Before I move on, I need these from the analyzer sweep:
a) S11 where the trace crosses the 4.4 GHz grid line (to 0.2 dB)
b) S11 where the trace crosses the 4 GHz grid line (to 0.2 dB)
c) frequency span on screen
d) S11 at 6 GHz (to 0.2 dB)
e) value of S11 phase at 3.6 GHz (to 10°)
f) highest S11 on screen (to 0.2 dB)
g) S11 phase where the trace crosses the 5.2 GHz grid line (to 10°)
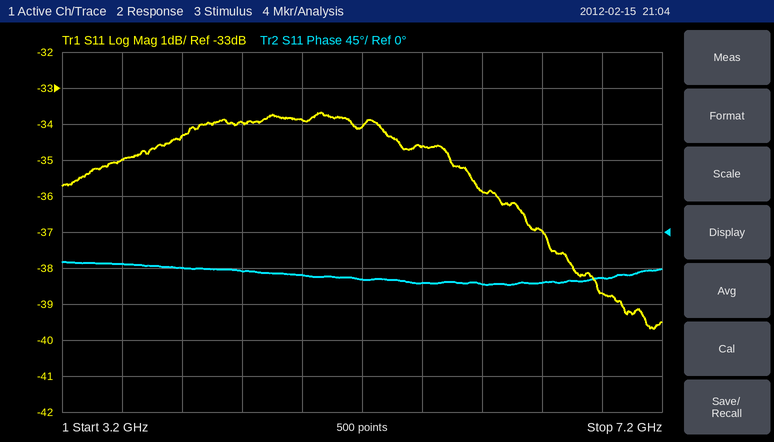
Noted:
-34.0 dB
-34.4 dB
4 GHz
-35.8 dB
-40°
-33.6 dB
-60°
